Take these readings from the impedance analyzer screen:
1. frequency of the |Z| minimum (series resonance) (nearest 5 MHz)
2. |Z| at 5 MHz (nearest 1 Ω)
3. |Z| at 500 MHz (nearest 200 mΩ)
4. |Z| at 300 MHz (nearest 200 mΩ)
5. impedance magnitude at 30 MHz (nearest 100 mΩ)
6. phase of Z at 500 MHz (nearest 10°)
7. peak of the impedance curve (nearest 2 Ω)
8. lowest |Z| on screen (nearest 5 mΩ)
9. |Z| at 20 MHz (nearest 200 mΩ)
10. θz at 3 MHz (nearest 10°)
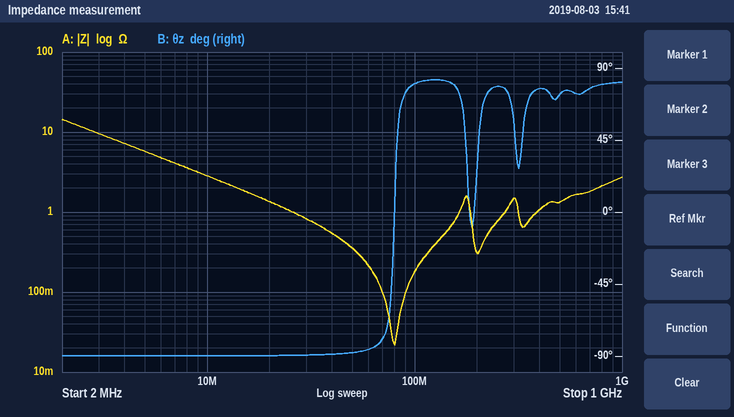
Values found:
80 MHz
6 Ω
1.4 Ω
1.4 Ω
800 mΩ
70°
14 Ω
20 mΩ
1.4 Ω
-90°
